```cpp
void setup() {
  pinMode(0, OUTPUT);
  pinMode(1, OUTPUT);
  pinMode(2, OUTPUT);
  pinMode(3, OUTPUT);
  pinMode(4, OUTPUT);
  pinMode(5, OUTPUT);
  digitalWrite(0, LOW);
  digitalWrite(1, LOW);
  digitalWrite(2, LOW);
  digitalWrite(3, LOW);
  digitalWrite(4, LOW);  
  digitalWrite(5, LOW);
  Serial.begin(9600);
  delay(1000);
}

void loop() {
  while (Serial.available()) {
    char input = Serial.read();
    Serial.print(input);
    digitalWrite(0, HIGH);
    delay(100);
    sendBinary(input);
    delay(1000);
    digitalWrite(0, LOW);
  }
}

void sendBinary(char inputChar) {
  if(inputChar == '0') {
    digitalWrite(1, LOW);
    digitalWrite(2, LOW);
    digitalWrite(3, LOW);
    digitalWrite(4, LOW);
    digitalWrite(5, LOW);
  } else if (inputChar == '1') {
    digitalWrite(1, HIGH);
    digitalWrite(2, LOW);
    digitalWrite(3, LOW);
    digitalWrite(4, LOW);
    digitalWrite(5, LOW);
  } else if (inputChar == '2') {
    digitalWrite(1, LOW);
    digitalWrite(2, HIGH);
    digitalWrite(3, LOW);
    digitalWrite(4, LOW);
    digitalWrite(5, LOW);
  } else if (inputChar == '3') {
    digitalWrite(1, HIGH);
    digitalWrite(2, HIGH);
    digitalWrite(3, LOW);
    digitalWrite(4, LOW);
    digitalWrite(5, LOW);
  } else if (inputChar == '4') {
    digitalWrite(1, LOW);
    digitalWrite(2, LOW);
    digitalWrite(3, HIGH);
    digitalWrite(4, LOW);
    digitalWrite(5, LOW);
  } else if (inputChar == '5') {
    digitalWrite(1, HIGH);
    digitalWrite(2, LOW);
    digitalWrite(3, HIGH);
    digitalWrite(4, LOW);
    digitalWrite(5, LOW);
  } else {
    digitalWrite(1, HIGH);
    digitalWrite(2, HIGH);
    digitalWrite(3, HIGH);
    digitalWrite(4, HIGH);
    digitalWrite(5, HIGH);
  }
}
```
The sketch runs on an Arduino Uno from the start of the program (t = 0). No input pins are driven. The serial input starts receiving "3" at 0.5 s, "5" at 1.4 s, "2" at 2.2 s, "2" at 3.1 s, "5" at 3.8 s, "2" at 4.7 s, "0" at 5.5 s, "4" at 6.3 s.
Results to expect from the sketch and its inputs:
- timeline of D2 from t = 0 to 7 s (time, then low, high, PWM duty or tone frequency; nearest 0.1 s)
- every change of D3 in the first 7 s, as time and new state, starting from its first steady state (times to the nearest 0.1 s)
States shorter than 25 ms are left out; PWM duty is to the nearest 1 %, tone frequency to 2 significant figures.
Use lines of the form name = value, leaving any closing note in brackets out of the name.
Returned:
timeline of D2 from t = 0 to 7 s = 0 s low; 1.1 s high; 2.2 s low; 3.3 s high; 5.5 s low; 6.6 s high
every change of D3 in the first 7 s, as time and new state, starting from its first steady state = 0 s low; 2.2 s high; 3.3 s low; 5.5 s high; 6.6 s low
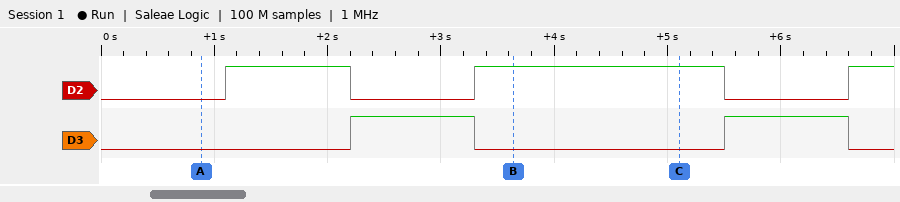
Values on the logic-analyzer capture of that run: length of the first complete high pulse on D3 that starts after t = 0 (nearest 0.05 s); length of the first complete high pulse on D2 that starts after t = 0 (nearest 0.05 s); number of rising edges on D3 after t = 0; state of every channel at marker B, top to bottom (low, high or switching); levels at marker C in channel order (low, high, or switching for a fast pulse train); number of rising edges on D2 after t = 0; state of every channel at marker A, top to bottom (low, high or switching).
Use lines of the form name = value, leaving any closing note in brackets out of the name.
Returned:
length of the first complete high pulse on D3 that starts after t = 0 = 1.10 s
length of the first complete high pulse on D2 that starts after t = 0 = 1.10 s
number of rising edges on D3 after t = 0 = 2
state of every channel at marker B, top to bottom = D2 high, D3 low
levels at marker C in channel order = D2 high, D3 low
number of rising edges on D2 after t = 0 = 3
state of every channel at marker A, top to bottom = D2 low, D3 low
